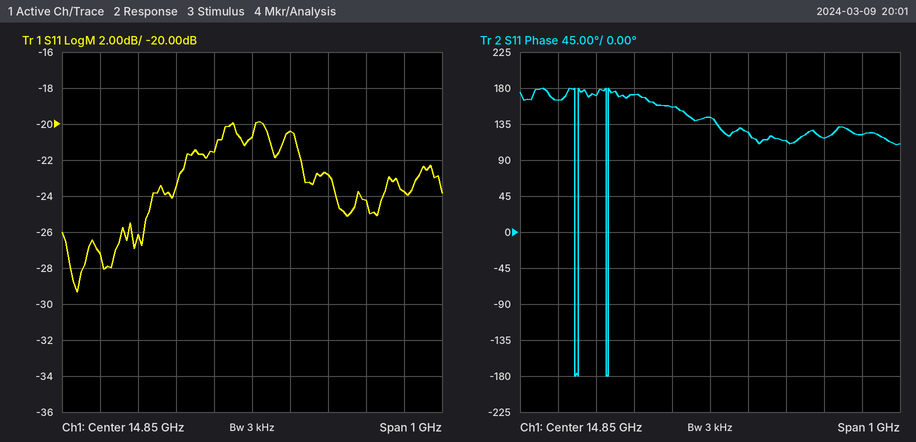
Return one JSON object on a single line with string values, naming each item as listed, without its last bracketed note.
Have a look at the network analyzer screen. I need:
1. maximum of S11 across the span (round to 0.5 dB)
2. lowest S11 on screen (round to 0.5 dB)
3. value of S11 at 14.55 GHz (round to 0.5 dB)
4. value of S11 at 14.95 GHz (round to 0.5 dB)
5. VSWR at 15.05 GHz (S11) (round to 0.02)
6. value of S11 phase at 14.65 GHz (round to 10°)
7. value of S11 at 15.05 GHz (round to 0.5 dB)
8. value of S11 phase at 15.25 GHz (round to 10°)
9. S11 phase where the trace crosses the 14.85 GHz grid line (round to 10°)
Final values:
{"maximum of S11 across the span": "-20.0 dB", "lowest S11 on screen": "-29.5 dB", "value of S11 at 14.55 GHz": "-26.0 dB", "value of S11 at 14.95 GHz": "-20.5 dB", "VSWR at 15.05 GHz (S11)": "1.16", "value of S11 phase at 14.65 GHz": "170°", "value of S11 at 15.05 GHz": "-23.0 dB", "value of S11 phase at 15.25 GHz": "120°", "S11 phase where the trace crosses the 14.85 GHz grid line": "140°"}
